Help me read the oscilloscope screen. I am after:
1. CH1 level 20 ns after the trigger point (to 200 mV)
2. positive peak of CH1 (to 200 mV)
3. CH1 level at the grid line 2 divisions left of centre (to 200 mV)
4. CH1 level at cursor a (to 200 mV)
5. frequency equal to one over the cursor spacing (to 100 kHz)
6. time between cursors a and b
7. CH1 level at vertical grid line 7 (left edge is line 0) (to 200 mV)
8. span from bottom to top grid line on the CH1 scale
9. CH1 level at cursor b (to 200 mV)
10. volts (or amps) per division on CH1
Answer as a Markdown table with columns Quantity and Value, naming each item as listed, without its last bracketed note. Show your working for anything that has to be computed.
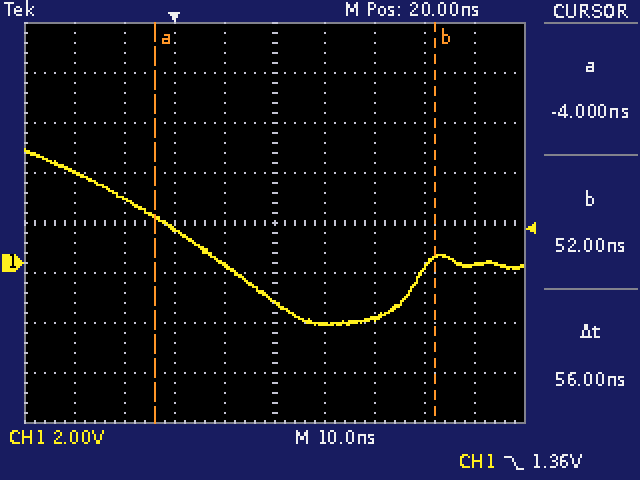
| Quantity | Value |
|---|---|
| CH1 level 20 ns after the trigger point | -1.6 V |
| positive peak of CH1 | 4.6 V |
| CH1 level at the grid line 2 divisions left of centre | 1.4 V |
| CH1 level at cursor a | 1.8 V |
| frequency equal to one over the cursor spacing | 1 / 56 ns ≈ 17.9 MHz |
| time between cursors a and b | 56 ns |
| CH1 level at vertical grid line 7 (left edge is line 0) | -2.2 V |
| span from bottom to top grid line on the CH1 scale | 16 V |
| CH1 level at cursor b | 200 mV |
| volts (or amps) per division on CH1 | 2 V |
